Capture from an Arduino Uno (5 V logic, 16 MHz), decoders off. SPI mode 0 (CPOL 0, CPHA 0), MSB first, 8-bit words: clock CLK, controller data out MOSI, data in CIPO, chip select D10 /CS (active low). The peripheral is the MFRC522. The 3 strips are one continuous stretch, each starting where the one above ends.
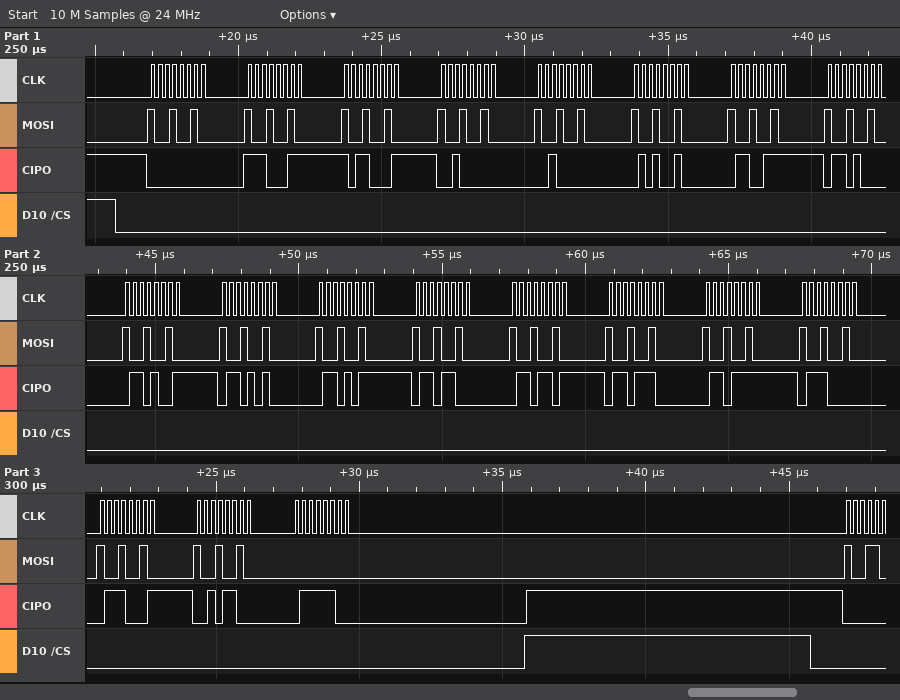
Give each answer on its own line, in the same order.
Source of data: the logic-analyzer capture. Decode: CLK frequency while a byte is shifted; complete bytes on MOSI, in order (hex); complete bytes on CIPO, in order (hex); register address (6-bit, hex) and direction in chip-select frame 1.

4 MHz
92 92 92 92 92 92 92 92 92 92 92 92 92 92 92 92 92 92 00
00 E3 B1 20 20 52 67 68 69 6A 6B 6C 6D 6E 6F 70 71 2C 7C
0x09 read
